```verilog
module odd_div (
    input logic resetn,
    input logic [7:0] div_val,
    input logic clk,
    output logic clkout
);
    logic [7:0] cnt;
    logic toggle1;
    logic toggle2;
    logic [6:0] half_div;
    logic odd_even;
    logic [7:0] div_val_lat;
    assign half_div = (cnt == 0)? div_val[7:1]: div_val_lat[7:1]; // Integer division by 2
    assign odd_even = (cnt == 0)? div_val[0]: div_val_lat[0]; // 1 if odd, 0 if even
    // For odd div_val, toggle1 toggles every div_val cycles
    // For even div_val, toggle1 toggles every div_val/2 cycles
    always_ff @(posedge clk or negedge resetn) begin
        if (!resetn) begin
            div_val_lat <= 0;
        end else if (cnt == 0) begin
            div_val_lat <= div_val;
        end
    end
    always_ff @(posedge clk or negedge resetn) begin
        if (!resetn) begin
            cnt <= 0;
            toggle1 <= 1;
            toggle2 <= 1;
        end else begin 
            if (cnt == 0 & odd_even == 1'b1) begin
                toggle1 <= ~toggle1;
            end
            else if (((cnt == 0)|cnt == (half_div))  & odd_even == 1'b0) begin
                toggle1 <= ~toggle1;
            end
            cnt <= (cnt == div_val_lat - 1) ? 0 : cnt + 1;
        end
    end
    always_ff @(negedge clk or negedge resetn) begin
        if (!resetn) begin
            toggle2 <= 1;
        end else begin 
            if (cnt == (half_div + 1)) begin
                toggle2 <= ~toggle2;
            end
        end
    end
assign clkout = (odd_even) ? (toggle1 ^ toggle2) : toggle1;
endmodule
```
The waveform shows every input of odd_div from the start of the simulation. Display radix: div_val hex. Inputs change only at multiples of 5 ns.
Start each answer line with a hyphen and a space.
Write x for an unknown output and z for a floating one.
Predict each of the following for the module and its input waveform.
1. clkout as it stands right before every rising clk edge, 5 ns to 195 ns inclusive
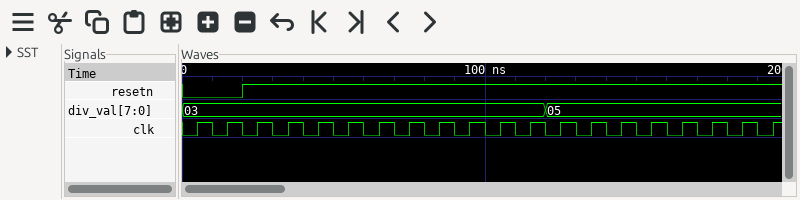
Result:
- 0 0 0 1 0 0 1 0 0 1 0 0 1 0 0 1 1 0 0 0
